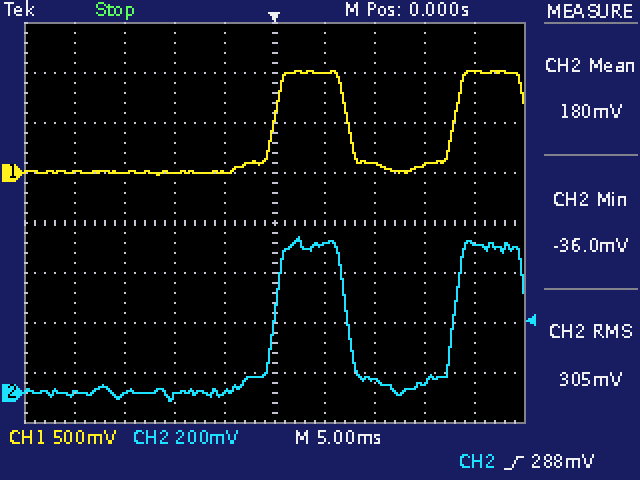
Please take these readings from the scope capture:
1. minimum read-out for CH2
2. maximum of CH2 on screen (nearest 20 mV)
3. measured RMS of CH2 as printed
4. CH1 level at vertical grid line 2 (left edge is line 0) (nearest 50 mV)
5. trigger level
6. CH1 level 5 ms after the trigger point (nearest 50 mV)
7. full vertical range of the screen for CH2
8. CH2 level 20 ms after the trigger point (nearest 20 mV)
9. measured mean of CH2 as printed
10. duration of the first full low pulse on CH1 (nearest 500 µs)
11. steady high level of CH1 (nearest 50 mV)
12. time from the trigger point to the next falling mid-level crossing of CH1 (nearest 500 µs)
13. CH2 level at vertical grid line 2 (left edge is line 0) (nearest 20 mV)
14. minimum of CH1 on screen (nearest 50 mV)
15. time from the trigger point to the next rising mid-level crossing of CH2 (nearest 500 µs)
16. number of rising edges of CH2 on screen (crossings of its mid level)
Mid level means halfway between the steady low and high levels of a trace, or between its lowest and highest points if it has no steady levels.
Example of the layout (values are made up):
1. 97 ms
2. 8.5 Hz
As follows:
1. -36.0 mV
2. 620 mV
3. 305 mV
4. 0 mV
5. 288 mV
6. 1.00 V
7. 1.6 V
8. 600 mV
9. 180 mV
10. 10.5 ms
11. 1.00 V
12. 7.5 ms
13. 0 mV
14. 0 mV
15. 18.0 ms
16. 2
